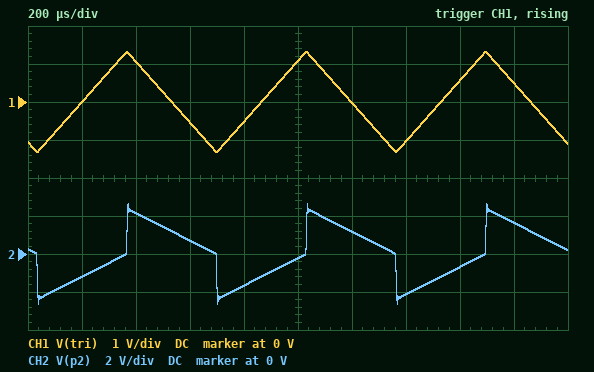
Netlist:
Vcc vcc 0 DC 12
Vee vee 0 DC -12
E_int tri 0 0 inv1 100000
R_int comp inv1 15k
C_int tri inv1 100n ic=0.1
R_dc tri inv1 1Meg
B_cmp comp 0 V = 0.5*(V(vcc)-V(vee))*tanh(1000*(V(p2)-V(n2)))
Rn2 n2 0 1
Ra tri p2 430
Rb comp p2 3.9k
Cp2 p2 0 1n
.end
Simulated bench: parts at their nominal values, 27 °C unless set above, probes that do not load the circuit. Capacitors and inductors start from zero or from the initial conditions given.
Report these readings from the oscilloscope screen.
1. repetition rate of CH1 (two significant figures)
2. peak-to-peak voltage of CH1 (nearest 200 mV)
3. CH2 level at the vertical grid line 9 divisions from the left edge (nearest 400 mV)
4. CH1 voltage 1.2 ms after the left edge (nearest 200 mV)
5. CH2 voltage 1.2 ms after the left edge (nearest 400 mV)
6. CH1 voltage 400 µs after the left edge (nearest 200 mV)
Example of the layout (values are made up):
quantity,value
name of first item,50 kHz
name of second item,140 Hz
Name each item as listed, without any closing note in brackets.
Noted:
quantity,value
repetition rate of CH1,1.5 kHz
peak-to-peak voltage of CH1,2.6 V
CH2 level at the vertical grid line 9 divisions from the left edge,1.6 V
CH1 voltage 1.2 ms after the left edge,0 V
CH2 voltage 1.2 ms after the left edge,1.2 V
CH1 voltage 400 µs after the left edge,1.0 V
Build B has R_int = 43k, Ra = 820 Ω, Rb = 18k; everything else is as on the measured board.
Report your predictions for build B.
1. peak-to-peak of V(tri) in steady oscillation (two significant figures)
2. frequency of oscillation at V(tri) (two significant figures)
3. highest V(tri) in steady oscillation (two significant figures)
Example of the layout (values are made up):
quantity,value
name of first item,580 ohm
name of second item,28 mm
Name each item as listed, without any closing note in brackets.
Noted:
quantity,value
peak-to-peak of V(tri) in steady oscillation,1.1 V
frequency of oscillation at V(tri),1.3 kHz
highest V(tri) in steady oscillation,540 mV
